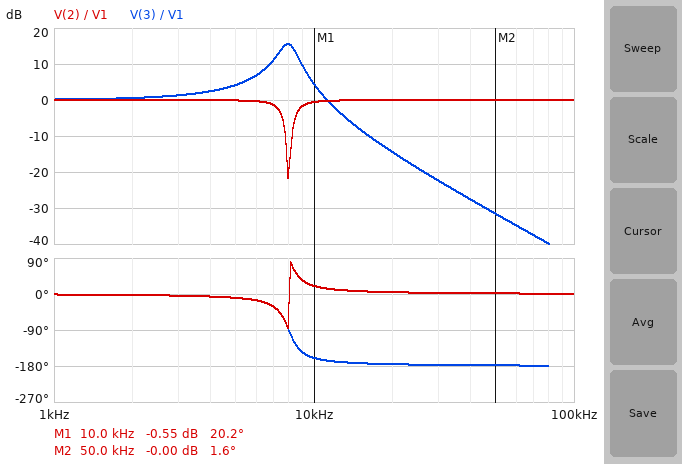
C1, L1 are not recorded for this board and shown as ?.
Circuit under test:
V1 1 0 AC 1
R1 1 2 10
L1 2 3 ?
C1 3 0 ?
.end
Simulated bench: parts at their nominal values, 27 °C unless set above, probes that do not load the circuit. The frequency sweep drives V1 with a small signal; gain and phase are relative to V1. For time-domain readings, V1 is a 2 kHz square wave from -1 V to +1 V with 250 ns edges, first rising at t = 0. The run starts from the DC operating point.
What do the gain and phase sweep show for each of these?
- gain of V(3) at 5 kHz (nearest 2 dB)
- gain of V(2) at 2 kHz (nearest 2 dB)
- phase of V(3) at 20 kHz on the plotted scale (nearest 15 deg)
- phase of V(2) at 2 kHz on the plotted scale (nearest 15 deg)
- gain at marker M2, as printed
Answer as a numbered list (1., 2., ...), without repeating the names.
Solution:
1. 4 dB
2. 0 dB
3. -180 deg
4. 0 deg
5. -0.00 dB
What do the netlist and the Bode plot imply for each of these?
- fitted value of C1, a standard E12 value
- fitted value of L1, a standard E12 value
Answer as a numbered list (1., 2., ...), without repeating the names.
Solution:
1. 330 nF
2. 1.2 mH
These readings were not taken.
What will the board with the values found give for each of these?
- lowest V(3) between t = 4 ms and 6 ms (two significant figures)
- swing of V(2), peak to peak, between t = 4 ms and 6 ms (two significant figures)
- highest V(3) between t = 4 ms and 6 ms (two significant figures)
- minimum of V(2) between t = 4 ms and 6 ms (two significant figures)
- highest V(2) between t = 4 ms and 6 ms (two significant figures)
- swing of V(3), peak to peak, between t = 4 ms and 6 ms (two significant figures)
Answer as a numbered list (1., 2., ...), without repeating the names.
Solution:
1. -2.1 V
2. 2.3 V
3. 2.1 V
4. -1.2 V
5. 1.2 V
6. 4.3 V
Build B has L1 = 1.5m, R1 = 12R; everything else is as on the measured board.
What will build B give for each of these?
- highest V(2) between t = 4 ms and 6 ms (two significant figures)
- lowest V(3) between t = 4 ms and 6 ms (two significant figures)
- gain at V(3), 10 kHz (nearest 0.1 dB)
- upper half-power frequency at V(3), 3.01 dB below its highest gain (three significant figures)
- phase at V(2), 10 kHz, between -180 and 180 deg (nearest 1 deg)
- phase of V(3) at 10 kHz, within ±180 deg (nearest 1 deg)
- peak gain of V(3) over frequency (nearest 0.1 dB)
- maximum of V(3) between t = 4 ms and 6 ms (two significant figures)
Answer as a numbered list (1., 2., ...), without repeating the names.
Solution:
1. 1.2 V
2. -2.4 V
3. 0.1 dB
4. 7.71 kHz
5. 15 deg
6. -165 deg
7. 15.0 dB
8. 2.4 V
